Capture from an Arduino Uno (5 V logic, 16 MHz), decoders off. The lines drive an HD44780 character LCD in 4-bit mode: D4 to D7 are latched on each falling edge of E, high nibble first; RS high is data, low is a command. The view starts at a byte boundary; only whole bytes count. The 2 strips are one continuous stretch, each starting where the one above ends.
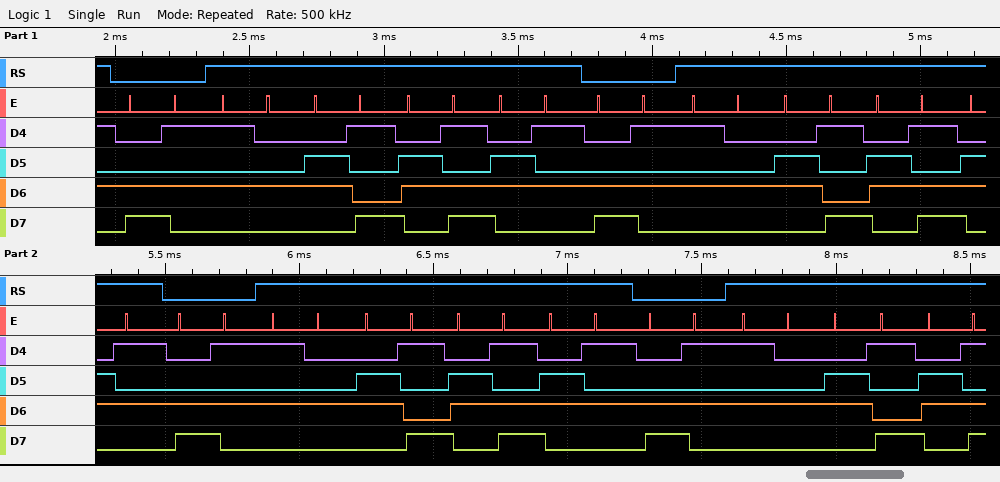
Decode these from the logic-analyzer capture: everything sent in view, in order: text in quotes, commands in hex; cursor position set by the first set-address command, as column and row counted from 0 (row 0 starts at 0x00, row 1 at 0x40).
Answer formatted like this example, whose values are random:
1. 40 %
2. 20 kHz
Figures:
1. 0xC5 "Time" 0xC5 "Time" 0xC5 "Time" 0xC5 "Tim"
2. column 5, row 1
